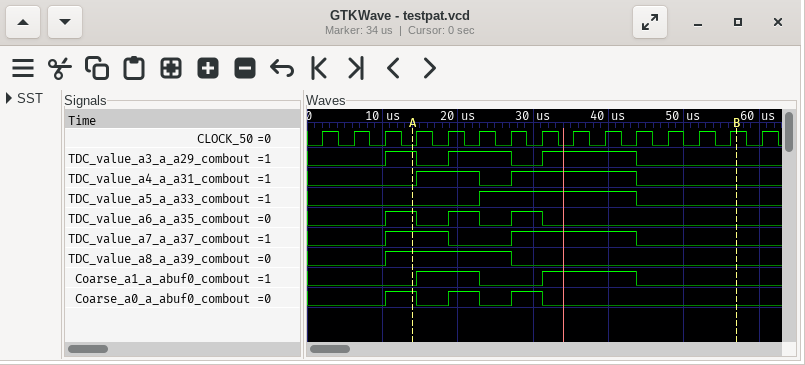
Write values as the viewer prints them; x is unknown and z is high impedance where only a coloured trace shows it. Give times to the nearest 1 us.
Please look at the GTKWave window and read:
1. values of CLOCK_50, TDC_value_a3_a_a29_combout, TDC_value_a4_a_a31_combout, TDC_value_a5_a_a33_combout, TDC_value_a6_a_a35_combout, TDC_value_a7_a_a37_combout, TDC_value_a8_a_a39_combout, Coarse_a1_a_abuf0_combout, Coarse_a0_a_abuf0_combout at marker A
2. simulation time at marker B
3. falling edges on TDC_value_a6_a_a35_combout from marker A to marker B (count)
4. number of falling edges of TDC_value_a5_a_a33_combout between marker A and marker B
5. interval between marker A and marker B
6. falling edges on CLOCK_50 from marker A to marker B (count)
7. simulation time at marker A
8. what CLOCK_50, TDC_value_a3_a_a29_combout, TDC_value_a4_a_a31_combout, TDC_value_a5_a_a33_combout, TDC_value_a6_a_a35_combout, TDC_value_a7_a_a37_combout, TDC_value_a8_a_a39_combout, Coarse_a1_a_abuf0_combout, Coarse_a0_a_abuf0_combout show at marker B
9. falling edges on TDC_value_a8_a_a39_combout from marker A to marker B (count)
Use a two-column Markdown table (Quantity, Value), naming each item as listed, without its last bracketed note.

| Quantity | Value |
|---|---|
| values of CLOCK_50, TDC_value_a3_a_a29_combout, TDC_value_a4_a_a31_combout, TDC_value_a5_a_a33_combout, TDC_value_a6_a_a35_combout, TDC_value_a7_a_a37_combout, TDC_value_a8_a_a39_combout, Coarse_a1_a_abuf0_combout, Coarse_a0_a_abuf0_combout at marker A | CLOCK_50=0, TDC_value_a3_a_a29_combout=1, TDC_value_a4_a_a31_combout=0, TDC_value_a5_a_a33_combout=0, TDC_value_a6_a_a35_combout=1, TDC_value_a7_a_a37_combout=1, TDC_value_a8_a_a39_combout=1, Coarse_a1_a_abuf0_combout=0, Coarse_a0_a_abuf0_combout=1 |
| simulation time at marker B | 57 us |
| falling edges on TDC_value_a6_a_a35_combout from marker A to marker B | 3 |
| number of falling edges of TDC_value_a5_a_a33_combout between marker A and marker B | 1 |
| interval between marker A and marker B | 43 us |
| falling edges on CLOCK_50 from marker A to marker B | 10 |
| simulation time at marker A | 14 us |
| what CLOCK_50, TDC_value_a3_a_a29_combout, TDC_value_a4_a_a31_combout, TDC_value_a5_a_a33_combout, TDC_value_a6_a_a35_combout, TDC_value_a7_a_a37_combout, TDC_value_a8_a_a39_combout, Coarse_a1_a_abuf0_combout, Coarse_a0_a_abuf0_combout show at marker B | CLOCK_50=1, TDC_value_a3_a_a29_combout=0, TDC_value_a4_a_a31_combout=0, TDC_value_a5_a_a33_combout=0, TDC_value_a6_a_a35_combout=0, TDC_value_a7_a_a37_combout=0, TDC_value_a8_a_a39_combout=0, Coarse_a1_a_abuf0_combout=0, Coarse_a0_a_abuf0_combout=0 |
| falling edges on TDC_value_a8_a_a39_combout from marker A to marker B | 1 |
